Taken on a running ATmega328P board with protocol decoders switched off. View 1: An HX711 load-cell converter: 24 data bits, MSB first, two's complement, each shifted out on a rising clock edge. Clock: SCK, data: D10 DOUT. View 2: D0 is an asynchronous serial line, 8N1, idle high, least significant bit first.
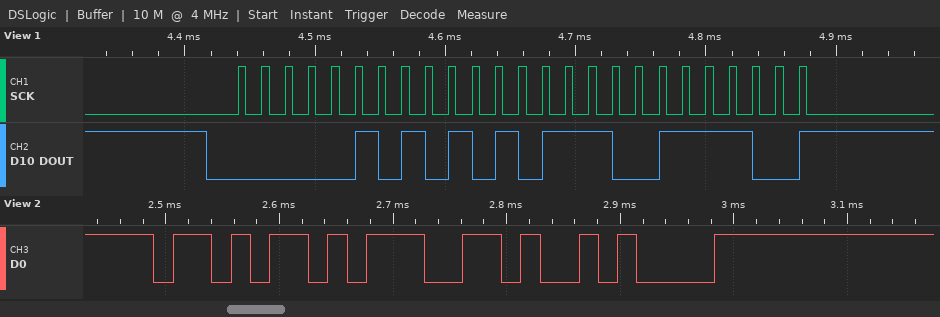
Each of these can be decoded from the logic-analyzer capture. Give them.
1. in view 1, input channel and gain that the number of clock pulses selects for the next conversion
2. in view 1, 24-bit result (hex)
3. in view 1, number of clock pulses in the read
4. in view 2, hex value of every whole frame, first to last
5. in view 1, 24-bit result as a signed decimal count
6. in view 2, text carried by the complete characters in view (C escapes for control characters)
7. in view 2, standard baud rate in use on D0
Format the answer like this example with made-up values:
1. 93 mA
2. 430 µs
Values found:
1. channel A, gain 128
2. 0x05573C
3. 25
4. 6B 67 0A
5. 350012
6. "kg\n"
7. 57600 baud
